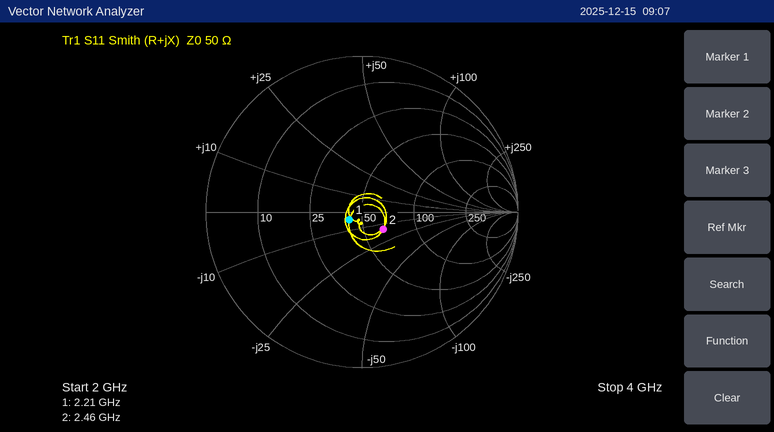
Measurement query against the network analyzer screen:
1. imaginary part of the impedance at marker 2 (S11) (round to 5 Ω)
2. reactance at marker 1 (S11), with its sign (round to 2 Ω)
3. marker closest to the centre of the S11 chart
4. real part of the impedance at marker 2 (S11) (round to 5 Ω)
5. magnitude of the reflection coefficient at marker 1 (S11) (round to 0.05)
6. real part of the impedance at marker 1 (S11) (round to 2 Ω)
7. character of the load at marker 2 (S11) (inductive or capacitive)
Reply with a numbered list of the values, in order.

1. -15 Ω
2. -4 Ω
3. marker 1
4. 65 Ω
5. 0.10
6. 42 Ω
7. capacitive
